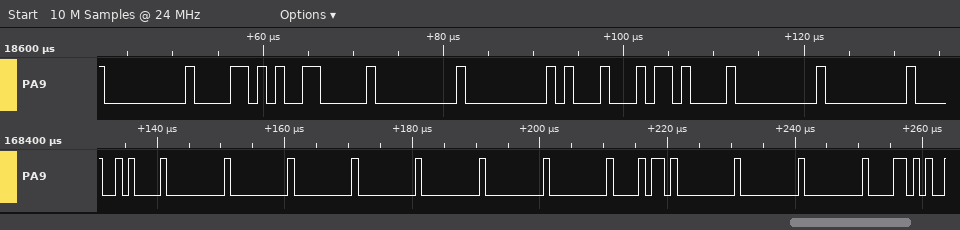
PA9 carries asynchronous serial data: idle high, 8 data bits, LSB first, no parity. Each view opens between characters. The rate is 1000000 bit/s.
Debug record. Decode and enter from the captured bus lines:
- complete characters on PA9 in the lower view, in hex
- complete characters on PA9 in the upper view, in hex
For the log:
0A, 00, 00, 00, 00, 00, 00, 00, 68, 00, 00, 00, 58
00, 58, 06, 00, 00, 11, 0B, 00, 00
